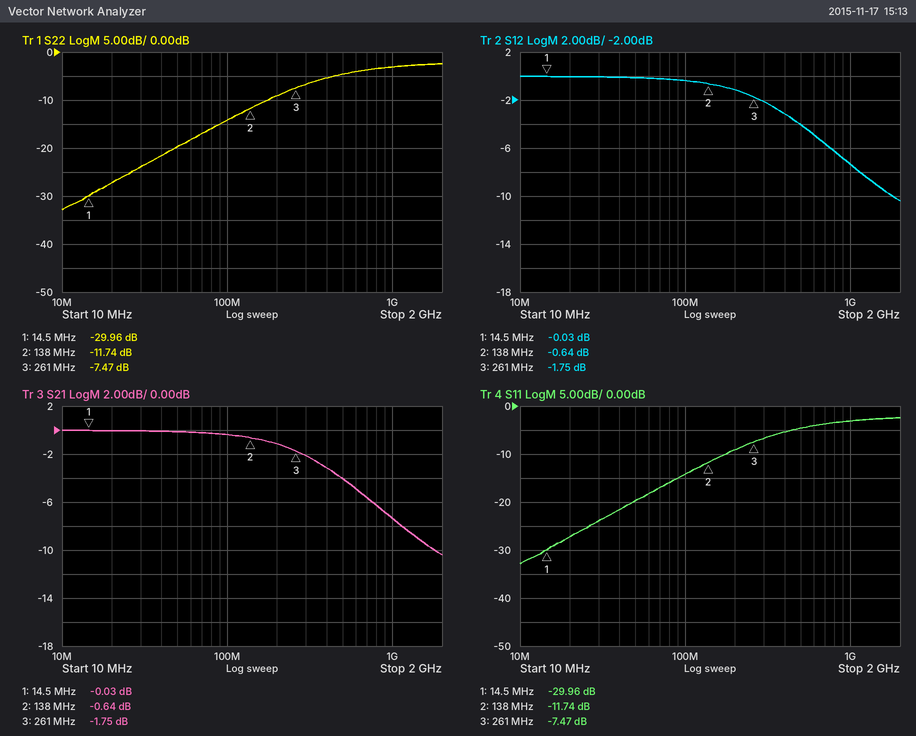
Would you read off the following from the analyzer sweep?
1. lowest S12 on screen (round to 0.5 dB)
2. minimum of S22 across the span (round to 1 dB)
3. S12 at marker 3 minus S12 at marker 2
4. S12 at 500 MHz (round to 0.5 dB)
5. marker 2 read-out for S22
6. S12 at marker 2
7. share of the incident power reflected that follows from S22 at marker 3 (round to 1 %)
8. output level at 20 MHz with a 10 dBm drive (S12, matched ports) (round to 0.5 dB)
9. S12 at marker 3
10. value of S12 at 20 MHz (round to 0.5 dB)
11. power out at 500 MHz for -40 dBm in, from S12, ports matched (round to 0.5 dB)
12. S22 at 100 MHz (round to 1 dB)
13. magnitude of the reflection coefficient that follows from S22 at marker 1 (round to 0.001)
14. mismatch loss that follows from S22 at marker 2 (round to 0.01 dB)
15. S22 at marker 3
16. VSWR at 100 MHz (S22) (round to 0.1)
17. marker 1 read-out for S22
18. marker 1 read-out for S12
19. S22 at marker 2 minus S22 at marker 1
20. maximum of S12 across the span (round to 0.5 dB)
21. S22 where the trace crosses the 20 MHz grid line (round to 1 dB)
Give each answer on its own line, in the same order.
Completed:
-10.5 dB
-33 dB
-1.11 dB
-4.0 dB
-11.74 dB
-0.64 dB
18 %
10.0 dBm
-1.75 dB
0.0 dB
-44.0 dBm
-14 dB
0.032
0.30 dB
-7.47 dB
1.5
-29.96 dB
-0.03 dB
18.22 dB
0.0 dB
-27 dB
